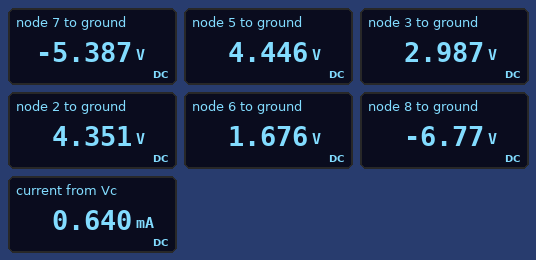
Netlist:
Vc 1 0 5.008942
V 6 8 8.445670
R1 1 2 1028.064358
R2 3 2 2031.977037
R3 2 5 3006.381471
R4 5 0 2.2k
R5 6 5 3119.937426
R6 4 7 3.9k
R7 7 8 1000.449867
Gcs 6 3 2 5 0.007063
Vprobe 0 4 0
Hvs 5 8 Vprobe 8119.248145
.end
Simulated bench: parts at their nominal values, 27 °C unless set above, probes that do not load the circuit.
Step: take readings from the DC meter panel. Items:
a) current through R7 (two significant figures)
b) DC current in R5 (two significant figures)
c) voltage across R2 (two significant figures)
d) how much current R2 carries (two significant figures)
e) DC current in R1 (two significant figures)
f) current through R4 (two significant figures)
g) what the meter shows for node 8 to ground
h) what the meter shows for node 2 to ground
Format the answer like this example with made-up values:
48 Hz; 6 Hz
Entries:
1.4 mA; 890 µA; 1.4 V; 670 µA; 640 µA; 2.0 mA; -6.77 V; 4.351 V
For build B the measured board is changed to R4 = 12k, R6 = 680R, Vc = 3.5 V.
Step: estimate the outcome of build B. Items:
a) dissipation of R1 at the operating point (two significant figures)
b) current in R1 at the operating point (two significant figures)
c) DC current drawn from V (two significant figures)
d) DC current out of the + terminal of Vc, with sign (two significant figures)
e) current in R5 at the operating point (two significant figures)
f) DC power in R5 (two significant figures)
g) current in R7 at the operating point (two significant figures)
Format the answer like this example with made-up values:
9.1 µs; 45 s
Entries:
74 µW; 270 µA; 1.5 mA; -270 µA; 1.2 mA; 4.5 mW; 580 µA
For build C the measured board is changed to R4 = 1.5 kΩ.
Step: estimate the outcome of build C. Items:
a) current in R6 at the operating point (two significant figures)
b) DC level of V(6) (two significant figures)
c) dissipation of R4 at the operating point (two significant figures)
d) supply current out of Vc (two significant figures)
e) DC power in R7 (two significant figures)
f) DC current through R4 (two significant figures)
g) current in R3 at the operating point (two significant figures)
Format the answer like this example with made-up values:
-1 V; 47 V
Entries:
1.2 mA; 2.6 V; 9.7 mW; 1.4 mA; 1.4 mW; 2.5 mA; 67 µA
